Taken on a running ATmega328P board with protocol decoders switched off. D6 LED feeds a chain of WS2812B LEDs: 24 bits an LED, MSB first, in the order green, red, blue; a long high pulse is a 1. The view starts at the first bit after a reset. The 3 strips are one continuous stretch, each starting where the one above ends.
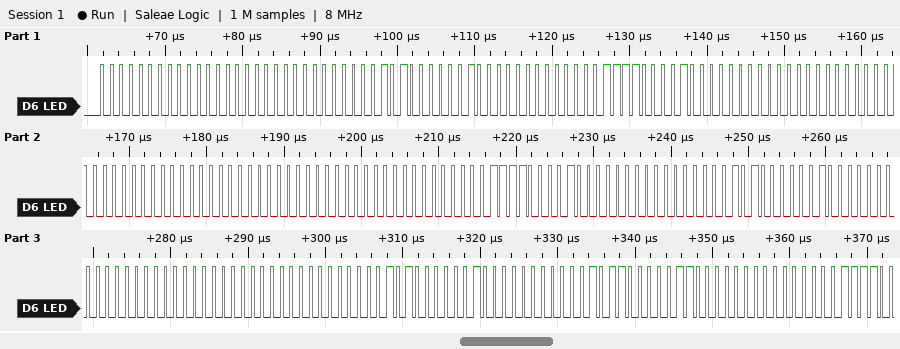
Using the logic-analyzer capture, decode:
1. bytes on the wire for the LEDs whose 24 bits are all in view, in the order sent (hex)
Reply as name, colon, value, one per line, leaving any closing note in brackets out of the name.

bytes on the wire for the LEDs whose 24 bits are all in view, in the order sent: 00 00 00 05 02 00 0F 08 00 00 00 00 00 00 00 0F 08 00 05 02 00 00 00 00 05 02 00 2C 18 00
